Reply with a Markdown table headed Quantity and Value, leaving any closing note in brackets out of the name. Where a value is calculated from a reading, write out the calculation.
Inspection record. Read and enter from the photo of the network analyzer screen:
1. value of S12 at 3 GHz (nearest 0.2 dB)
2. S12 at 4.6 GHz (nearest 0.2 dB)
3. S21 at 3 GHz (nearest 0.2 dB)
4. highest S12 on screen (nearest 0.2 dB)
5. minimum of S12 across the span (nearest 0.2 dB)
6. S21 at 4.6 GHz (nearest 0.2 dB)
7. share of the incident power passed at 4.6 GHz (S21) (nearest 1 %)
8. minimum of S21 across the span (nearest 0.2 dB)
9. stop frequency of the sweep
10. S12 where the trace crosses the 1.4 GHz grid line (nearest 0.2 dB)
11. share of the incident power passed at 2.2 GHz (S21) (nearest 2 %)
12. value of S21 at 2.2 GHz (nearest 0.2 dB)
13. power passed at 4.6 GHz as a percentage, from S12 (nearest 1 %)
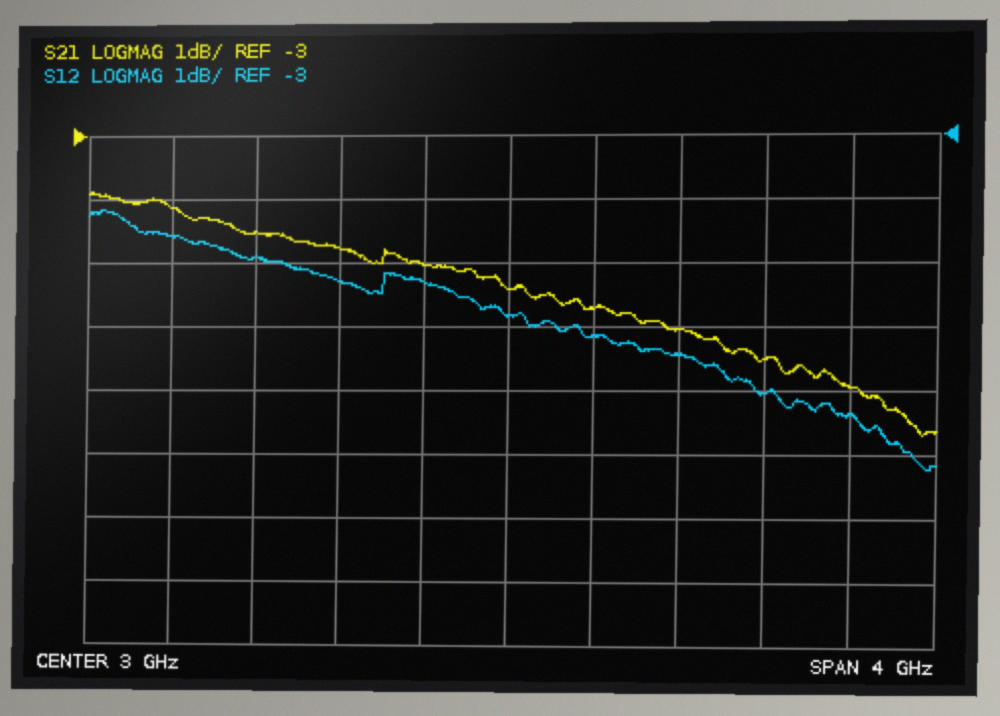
| Quantity | Value |
|---|---|
| value of S12 at 3 GHz | -5.8 dB |
| S12 at 4.6 GHz | -7.4 dB |
| S21 at 3 GHz | -5.4 dB |
| highest S12 on screen | -4.2 dB |
| minimum of S12 across the span | -8.2 dB |
| S21 at 4.6 GHz | -7.0 dB |
| share of the incident power passed at 4.6 GHz (S21) | 10^(-7/10) ≈ 20 % |
| minimum of S21 across the span | -7.6 dB |
| stop frequency of the sweep | 5 GHz |
| S12 where the trace crosses the 1.4 GHz grid line | -4.6 dB |
| share of the incident power passed at 2.2 GHz (S21) | 10^(-4.8/10) ≈ 33.1 %, so 34 % to the nearest 2 % |
| value of S21 at 2.2 GHz | -4.8 dB |
| power passed at 4.6 GHz as a percentage, from S12 | 10^(-7.4/10) ≈ 18 % |
